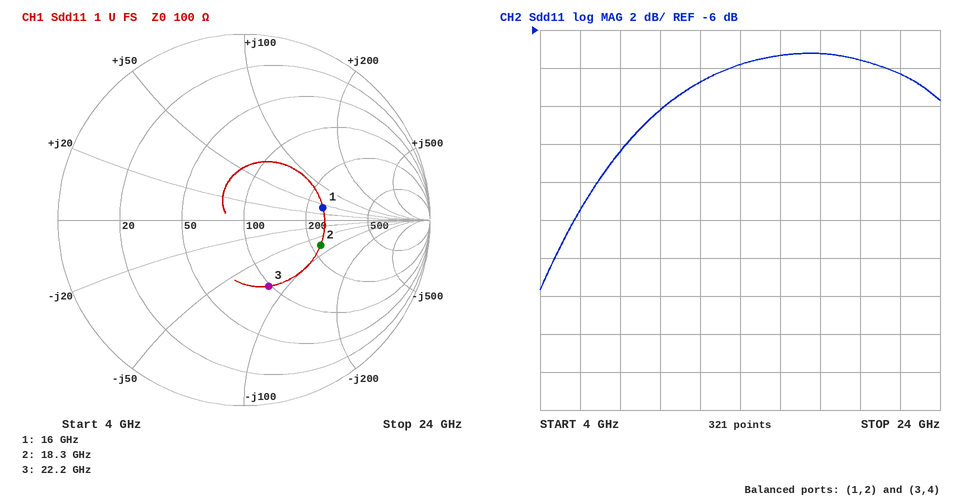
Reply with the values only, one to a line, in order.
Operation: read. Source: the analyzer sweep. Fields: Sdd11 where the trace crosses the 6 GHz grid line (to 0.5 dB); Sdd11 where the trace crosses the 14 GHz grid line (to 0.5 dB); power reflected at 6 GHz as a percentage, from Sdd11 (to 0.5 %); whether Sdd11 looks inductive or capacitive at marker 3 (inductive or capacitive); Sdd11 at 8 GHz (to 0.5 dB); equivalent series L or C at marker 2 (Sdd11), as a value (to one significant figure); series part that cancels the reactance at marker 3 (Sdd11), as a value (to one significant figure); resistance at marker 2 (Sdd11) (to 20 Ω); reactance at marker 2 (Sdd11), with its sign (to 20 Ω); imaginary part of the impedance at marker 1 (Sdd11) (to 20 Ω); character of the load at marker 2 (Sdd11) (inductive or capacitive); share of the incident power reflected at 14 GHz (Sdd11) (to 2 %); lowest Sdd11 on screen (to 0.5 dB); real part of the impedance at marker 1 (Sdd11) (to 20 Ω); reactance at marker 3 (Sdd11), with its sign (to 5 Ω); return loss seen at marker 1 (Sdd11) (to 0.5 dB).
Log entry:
-15.5 dB
-8.0 dB
3.0 %
capacitive
-12.5 dB
100 fF
600 pH
220 Ω
-80 Ω
+40 Ω
capacitive
16 %
-19.5 dB
240 Ω
-80 Ω
7.5 dB
